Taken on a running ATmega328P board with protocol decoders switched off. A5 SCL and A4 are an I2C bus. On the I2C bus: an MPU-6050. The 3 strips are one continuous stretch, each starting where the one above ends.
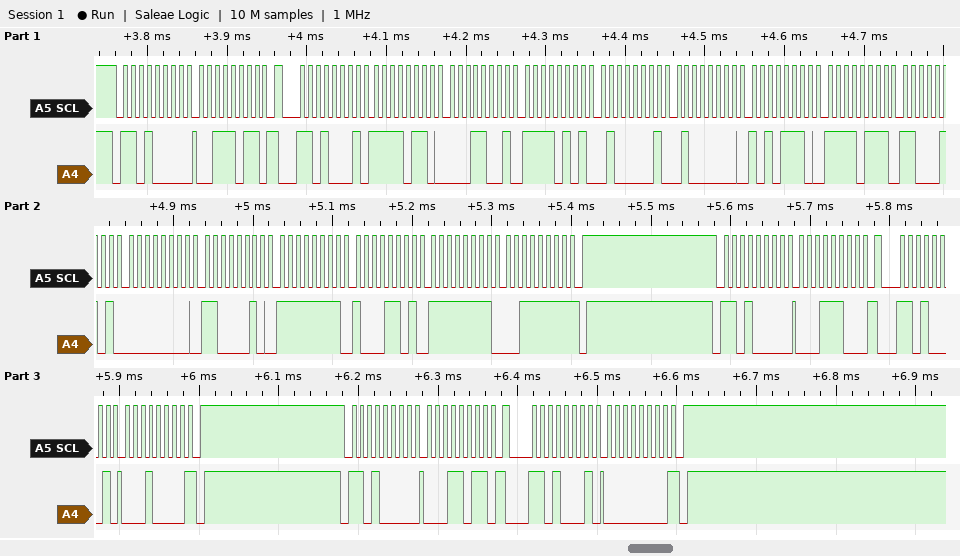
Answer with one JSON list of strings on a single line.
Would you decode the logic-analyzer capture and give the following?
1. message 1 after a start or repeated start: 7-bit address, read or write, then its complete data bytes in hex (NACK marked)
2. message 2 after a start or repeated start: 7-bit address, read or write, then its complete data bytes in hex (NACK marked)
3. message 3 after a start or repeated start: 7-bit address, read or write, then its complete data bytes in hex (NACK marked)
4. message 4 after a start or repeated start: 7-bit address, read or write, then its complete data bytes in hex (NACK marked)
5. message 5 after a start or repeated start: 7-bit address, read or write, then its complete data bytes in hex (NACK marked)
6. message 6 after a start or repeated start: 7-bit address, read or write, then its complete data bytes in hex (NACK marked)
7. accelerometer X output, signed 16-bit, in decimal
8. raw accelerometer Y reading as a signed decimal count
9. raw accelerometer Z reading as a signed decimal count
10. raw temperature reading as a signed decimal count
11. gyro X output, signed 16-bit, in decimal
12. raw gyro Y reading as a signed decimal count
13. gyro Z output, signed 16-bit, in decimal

["0x68 write: 3B", "0x68 read: F6 19 F5 41 40 AE F7 C5 00 C2 FF 8D FF 3F NACK", "0x68 write: 1C", "0x68 read: 10 NACK", "0x68 write: 1B", "0x68 read: 00 NACK", "-2535", "-2751", "16558", "-2107", "194", "-115", "-193"]
